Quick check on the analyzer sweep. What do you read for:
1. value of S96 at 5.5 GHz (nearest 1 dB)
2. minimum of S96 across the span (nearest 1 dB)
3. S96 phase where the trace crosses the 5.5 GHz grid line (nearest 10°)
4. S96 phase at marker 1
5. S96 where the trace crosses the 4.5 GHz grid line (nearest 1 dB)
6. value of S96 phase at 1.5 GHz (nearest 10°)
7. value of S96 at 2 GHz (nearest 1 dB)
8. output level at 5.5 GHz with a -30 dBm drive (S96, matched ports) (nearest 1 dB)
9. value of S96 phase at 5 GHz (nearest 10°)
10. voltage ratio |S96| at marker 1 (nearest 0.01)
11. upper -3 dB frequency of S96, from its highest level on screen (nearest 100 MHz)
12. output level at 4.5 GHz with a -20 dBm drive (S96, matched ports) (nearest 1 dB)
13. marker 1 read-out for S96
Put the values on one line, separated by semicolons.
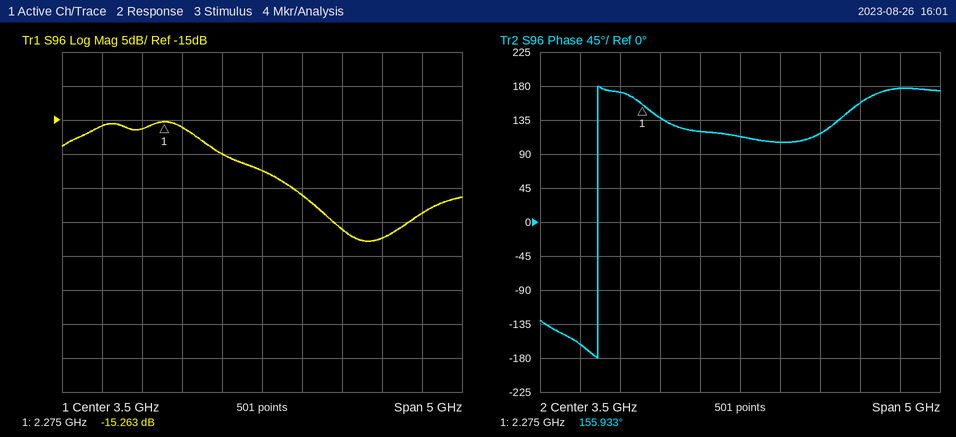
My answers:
-29 dB; -33 dB; 180°; 155.933°; -31 dB; -160°; -16 dB; -59 dBm; 160°; 0.17; 2.8 GHz; -51 dBm; -15.263 dB
